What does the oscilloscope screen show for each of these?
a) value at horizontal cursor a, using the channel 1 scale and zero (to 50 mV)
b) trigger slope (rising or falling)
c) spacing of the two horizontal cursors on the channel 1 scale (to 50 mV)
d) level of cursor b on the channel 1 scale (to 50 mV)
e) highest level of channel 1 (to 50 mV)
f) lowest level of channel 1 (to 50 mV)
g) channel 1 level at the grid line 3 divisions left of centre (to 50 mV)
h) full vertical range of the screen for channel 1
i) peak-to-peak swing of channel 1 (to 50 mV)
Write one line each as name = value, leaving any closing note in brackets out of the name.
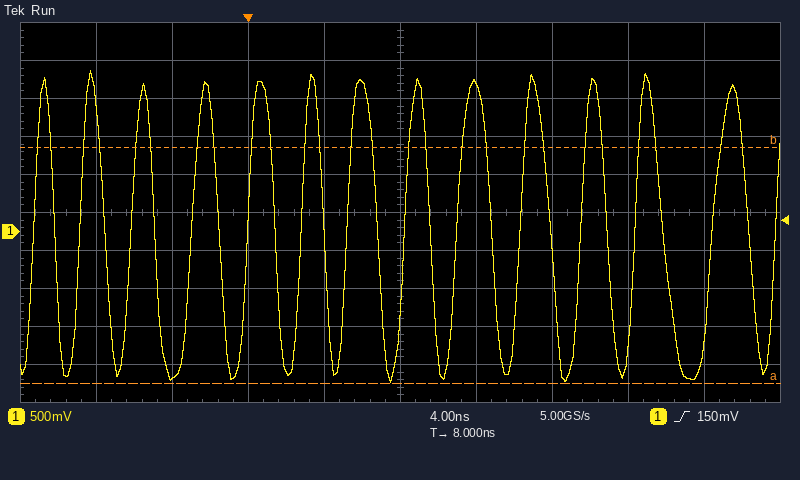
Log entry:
value at horizontal cursor a, using the channel 1 scale and zero = -2.00 V
trigger slope = rising
spacing of the two horizontal cursors on the channel 1 scale = 3.10 V
level of cursor b on the channel 1 scale = 1.10 V
highest level of channel 1 = 2.10 V
lowest level of channel 1 = -2.00 V
channel 1 level at the grid line 3 divisions left of centre = -1.90 V
full vertical range of the screen for channel 1 = 5 V
peak-to-peak swing of channel 1 = 4.10 V
